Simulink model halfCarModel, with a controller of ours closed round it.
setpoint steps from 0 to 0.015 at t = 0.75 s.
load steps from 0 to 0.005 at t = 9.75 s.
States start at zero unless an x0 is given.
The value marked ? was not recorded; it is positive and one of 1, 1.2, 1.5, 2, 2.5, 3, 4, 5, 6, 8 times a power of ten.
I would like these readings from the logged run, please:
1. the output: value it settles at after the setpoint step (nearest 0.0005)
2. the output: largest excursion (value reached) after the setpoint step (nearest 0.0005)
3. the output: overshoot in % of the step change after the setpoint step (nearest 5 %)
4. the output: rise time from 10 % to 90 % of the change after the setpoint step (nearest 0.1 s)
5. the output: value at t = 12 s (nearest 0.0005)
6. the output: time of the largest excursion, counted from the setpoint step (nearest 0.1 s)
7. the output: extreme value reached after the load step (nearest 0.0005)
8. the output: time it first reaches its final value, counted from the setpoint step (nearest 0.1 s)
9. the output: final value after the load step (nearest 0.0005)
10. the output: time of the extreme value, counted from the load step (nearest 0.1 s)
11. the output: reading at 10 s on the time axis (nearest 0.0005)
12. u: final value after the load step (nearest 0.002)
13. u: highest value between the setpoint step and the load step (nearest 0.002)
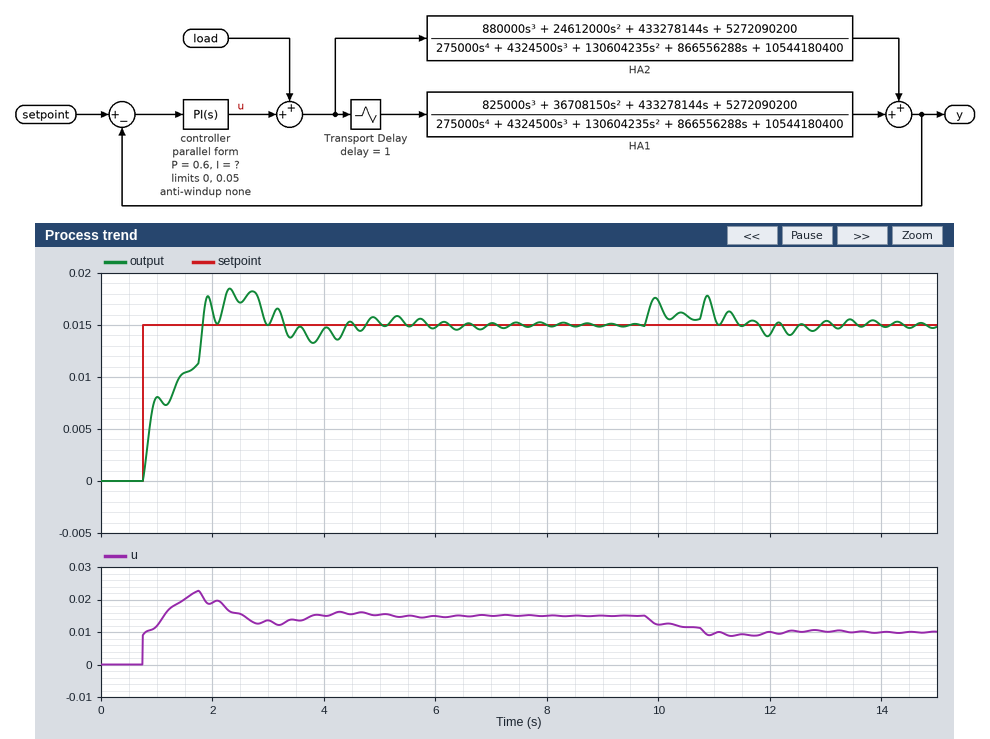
0.0150
0.0185
25 %
1.0 s
0.0140
1.6 s
0.0180
1.1 s
0.0150
1.1 s
0.0175
0.010
0.022
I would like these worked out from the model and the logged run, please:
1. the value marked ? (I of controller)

3
